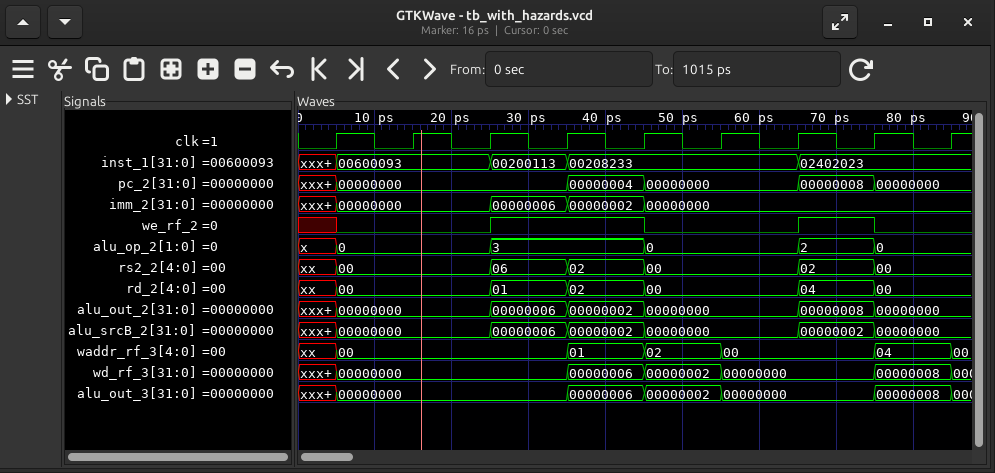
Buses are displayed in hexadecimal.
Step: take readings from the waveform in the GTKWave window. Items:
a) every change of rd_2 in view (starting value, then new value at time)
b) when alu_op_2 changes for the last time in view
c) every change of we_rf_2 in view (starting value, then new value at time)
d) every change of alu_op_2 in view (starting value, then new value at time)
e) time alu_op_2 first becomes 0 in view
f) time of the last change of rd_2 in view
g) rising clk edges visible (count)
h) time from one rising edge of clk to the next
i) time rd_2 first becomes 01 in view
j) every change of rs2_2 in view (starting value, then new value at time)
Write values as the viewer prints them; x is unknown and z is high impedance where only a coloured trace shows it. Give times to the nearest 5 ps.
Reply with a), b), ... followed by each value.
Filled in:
a) xx, 00 at 5 ps, 01 at 25 ps, 02 at 35 ps, 00 at 45 ps, 04 at 65 ps, 00 at 75 ps
b) 75 ps
c) x, 0 at 5 ps, 1 at 25 ps, 0 at 45 ps, 1 at 65 ps, 0 at 75 ps
d) x, 0 at 5 ps, 3 at 25 ps, 0 at 45 ps, 2 at 65 ps, 0 at 75 ps
e) 5 ps
f) 75 ps
g) 9
h) 10 ps
i) 25 ps
j) xx, 00 at 5 ps, 06 at 25 ps, 02 at 35 ps, 00 at 45 ps, 02 at 65 ps, 00 at 75 ps
